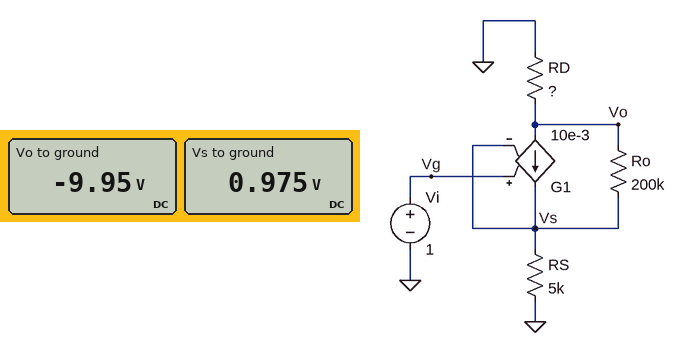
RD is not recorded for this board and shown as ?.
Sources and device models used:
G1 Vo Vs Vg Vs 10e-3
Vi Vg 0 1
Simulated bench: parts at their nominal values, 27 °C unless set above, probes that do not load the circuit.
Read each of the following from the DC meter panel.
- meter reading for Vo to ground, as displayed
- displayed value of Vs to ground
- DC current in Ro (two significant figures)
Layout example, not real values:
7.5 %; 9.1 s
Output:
-9.95 V; 0.975 V; 55 µA
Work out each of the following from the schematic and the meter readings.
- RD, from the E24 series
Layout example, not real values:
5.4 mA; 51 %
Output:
51 kΩ
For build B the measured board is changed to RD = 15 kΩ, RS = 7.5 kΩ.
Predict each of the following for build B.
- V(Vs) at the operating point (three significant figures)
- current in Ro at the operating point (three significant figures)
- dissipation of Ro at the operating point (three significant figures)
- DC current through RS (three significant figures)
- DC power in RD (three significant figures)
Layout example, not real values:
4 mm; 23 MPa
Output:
985 mV; 14.8 µA; 43.7 µW; 131 µA; 259 µW
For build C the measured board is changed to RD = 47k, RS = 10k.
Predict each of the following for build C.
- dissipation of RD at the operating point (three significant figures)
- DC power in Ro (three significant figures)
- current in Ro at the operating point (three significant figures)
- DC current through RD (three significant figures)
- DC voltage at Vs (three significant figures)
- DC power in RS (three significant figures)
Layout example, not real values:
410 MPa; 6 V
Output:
458 µW; 158 µW; 28.1 µA; 98.7 µA; 987 mV; 97.5 µW
